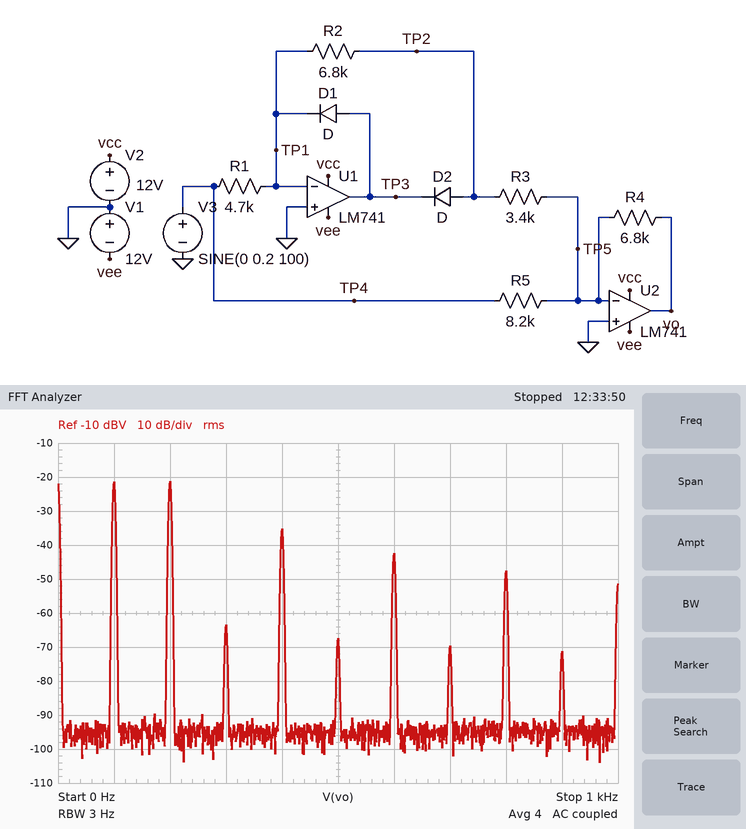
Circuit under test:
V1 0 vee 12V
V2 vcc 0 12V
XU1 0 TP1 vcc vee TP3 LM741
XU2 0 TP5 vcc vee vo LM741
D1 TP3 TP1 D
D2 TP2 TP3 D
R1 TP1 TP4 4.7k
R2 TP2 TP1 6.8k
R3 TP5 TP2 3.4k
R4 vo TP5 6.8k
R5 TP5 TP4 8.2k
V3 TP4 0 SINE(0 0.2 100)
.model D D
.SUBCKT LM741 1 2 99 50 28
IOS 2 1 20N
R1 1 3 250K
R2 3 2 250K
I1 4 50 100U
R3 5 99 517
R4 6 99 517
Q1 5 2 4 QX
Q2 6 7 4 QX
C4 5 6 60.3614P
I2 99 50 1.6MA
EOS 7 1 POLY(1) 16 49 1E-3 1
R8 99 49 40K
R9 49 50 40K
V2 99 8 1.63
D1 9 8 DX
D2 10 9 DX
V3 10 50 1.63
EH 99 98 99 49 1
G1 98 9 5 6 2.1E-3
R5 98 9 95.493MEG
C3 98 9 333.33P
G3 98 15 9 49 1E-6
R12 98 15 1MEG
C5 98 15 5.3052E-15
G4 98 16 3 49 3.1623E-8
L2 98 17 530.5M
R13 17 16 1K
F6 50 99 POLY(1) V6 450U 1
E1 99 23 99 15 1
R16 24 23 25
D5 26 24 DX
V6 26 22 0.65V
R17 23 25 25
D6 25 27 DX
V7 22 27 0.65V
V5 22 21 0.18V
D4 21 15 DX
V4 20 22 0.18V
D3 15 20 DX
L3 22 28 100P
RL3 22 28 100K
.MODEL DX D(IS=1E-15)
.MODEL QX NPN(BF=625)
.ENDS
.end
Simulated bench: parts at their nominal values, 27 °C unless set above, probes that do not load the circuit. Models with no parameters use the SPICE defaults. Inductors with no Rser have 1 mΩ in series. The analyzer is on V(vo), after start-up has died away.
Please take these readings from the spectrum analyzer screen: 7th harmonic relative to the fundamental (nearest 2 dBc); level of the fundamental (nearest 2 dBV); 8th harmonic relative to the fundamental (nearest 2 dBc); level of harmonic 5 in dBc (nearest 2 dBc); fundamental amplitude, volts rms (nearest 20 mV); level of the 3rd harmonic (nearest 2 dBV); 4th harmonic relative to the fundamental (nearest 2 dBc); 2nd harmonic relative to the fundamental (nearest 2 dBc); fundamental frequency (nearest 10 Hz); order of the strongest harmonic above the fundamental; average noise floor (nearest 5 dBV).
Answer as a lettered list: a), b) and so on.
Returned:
a) -48 dBc
b) -22 dBV
c) -26 dBc
d) -46 dBc
e) 80 mV
f) -64 dBV
g) -14 dBc
h) 0 dBc
i) 100 Hz
j) 2
k) -95 dBV
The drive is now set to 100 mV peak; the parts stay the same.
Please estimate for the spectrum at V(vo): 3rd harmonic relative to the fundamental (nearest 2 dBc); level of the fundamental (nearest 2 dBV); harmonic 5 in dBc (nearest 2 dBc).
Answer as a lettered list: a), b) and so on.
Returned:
a) -36 dBc
b) -28 dBV
c) -40 dBc
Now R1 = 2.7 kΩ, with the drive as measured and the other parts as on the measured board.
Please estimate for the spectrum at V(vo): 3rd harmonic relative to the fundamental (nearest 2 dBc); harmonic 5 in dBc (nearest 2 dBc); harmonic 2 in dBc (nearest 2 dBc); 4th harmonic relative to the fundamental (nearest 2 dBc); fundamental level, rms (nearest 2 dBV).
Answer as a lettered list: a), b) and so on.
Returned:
a) -48 dBc
b) -52 dBc
c) -4 dBc
d) -18 dBc
e) -12 dBV
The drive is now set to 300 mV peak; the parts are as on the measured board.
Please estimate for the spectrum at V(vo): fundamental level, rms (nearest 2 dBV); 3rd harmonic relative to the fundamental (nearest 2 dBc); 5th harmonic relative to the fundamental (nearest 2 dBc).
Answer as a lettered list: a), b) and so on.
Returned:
a) -18 dBV
b) -46 dBc
c) -50 dBc
